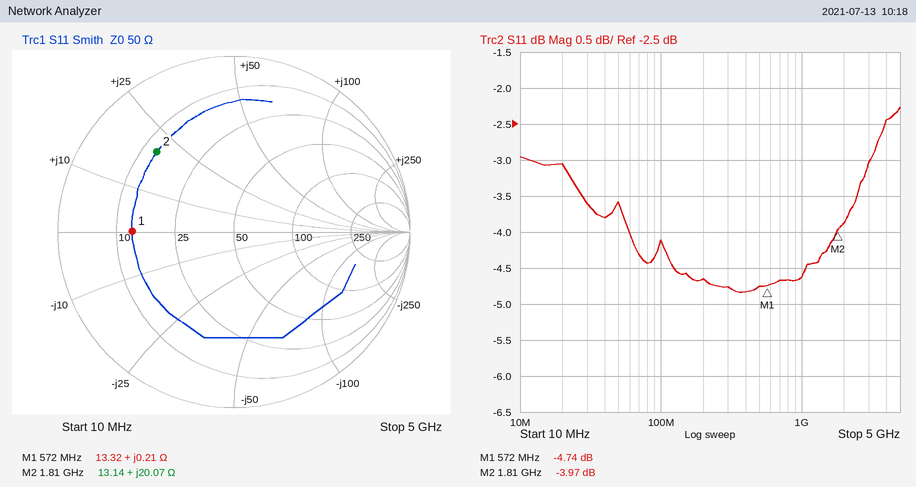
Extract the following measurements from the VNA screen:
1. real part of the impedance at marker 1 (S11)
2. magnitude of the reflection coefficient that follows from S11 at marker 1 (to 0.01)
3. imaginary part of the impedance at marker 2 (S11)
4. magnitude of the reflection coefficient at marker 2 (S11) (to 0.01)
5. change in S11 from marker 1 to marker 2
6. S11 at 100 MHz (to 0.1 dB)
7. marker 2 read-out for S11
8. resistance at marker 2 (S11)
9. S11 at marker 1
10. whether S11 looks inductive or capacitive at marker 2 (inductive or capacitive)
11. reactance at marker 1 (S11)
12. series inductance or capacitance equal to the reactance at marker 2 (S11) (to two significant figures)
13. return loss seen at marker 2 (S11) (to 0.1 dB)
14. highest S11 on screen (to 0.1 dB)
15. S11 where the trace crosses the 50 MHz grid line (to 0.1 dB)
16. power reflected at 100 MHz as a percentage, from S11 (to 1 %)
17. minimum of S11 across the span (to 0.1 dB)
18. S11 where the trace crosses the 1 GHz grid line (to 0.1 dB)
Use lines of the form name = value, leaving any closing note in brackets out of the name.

real part of the impedance at marker 1 = 13.32 Ω
magnitude of the reflection coefficient that follows from S11 at marker 1 = 0.58
imaginary part of the impedance at marker 2 = +20.07 Ω
magnitude of the reflection coefficient at marker 2 (S11) = 0.63
change in S11 from marker 1 to marker 2 = 0.77 dB
S11 at 100 MHz = -4.1 dB
marker 2 read-out for S11 = -3.97 dB
resistance at marker 2 = 13.14 Ω
S11 at marker 1 = -4.74 dB
whether S11 looks inductive or capacitive at marker 2 = inductive
reactance at marker 1 = +0.21 Ω
series inductance or capacitance equal to the reactance at marker 2 (S11) = 1.8 nH
return loss seen at marker 2 (S11) = 4.0 dB
highest S11 on screen = -2.3 dB
S11 where the trace crosses the 50 MHz grid line = -3.6 dB
power reflected at 100 MHz as a percentage, from S11 = 39 %
minimum of S11 across the span = -4.8 dB
S11 where the trace crosses the 1 GHz grid line = -4.6 dB
